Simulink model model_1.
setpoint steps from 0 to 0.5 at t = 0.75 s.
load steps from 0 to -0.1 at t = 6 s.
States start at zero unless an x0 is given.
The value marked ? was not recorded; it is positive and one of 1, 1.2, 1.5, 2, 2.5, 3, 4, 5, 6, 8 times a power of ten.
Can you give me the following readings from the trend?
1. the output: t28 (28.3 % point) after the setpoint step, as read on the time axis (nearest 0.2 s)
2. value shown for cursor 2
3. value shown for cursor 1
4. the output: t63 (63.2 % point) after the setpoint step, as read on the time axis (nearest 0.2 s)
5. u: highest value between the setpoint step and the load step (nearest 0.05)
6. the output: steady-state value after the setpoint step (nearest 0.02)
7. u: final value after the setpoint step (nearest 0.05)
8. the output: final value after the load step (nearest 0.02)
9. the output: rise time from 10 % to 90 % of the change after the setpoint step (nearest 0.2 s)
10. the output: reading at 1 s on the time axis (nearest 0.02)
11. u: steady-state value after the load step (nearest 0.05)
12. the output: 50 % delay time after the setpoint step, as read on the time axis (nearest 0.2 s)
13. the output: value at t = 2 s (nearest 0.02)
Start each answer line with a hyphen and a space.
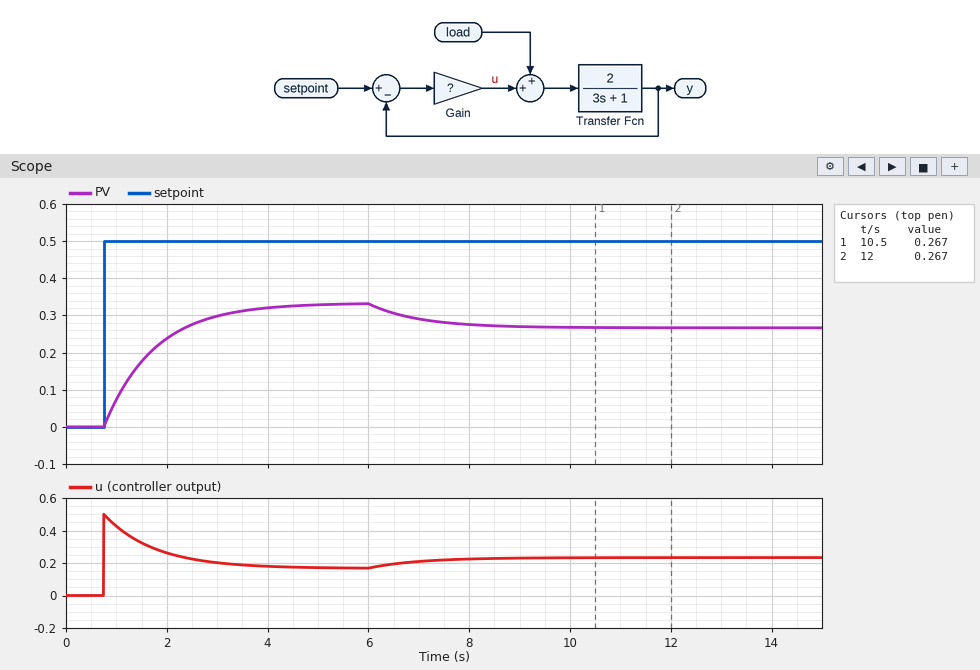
- 1.0 s
- 0.267
- 0.267
- 1.8 s
- 0.50
- 0.34
- 0.15
- 0.26
- 2.2 s
- 0.08
- 0.25
- 1.4 s
- 0.24
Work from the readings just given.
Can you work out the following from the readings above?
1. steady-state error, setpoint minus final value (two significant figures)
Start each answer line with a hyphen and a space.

- 0.16
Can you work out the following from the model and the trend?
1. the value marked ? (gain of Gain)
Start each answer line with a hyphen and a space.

- 1
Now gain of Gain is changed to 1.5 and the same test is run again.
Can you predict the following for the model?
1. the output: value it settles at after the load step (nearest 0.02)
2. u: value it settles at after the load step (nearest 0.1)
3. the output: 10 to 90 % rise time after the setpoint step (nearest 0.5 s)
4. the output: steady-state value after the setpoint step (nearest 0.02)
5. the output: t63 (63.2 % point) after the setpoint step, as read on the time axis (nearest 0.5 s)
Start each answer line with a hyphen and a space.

- 0.32
- 0.3
- 1.5 s
- 0.38
- 1.5 s
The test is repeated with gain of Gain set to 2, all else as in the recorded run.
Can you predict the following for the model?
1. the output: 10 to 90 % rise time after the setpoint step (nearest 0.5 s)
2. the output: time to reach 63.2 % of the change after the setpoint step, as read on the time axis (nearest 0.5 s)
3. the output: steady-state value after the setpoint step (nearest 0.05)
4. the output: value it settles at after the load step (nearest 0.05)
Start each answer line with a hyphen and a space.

- 1.5 s
- 1.5 s
- 0.40
- 0.35
